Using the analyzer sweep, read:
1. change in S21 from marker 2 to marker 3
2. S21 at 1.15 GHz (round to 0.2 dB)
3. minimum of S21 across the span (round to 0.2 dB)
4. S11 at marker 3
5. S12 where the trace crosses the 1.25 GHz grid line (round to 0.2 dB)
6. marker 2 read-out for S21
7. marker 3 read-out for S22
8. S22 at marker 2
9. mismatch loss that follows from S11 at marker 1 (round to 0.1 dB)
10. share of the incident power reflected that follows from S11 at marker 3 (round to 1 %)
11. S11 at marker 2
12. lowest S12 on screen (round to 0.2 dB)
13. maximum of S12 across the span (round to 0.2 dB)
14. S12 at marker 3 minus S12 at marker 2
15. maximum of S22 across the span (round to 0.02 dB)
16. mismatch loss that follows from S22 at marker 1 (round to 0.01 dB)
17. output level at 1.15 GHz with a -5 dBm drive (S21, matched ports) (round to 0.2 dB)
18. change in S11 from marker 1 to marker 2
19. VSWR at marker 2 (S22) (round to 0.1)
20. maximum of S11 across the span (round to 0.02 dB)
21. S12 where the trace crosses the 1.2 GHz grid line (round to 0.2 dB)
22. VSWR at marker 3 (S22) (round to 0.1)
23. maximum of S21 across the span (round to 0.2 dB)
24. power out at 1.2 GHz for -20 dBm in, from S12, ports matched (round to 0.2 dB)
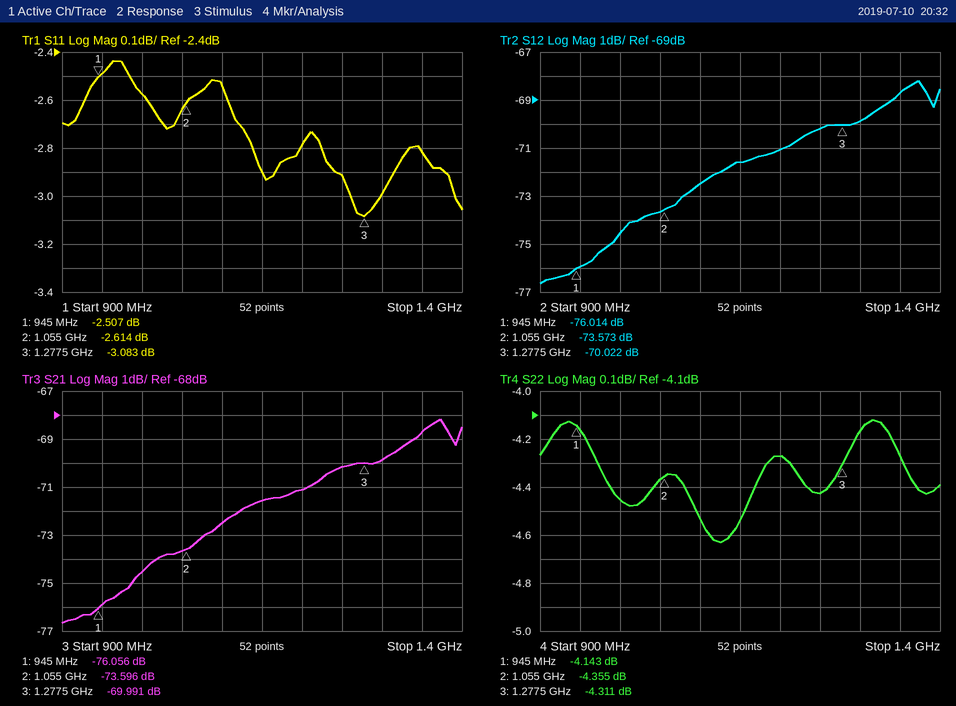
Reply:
3.605 dB
-71.6 dB
-76.6 dB
-3.083 dB
-70.2 dB
-73.596 dB
-4.311 dB
-4.355 dB
3.6 dB
49 %
-2.614 dB
-76.6 dB
-68.2 dB
3.551 dB
-4.12 dB
2.11 dB
-76.6 dBm
-0.107 dB
4.1
-2.44 dB
-71.0 dB
4.1
-68.2 dB
-91.0 dBm
